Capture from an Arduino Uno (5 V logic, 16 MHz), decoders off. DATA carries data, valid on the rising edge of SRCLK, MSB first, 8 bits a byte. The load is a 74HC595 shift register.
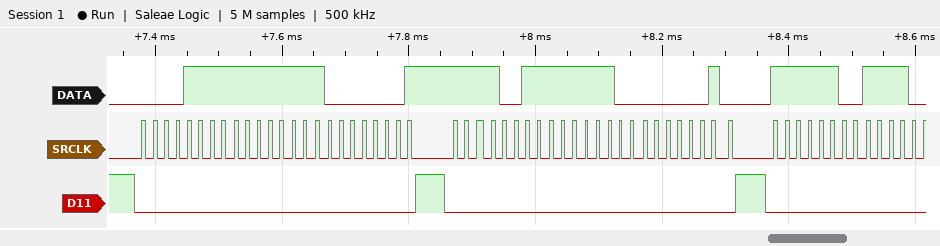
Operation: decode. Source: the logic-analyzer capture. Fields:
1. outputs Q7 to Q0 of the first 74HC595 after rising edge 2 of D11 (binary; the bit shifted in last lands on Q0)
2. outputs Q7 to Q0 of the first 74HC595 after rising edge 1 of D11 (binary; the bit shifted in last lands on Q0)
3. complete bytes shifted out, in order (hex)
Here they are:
00000010
00000001
0F FF 01 F3 FC 02 FC
